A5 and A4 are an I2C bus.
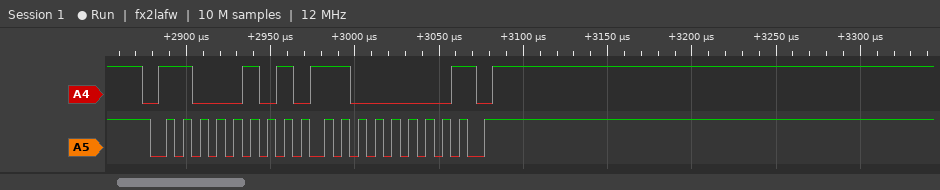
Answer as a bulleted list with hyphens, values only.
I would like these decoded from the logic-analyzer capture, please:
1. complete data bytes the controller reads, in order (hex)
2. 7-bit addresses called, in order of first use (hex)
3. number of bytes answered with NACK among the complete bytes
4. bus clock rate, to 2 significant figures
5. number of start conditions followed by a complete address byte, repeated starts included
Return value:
- C0
- 0x62
- 1
- 100 kHz
- 1
